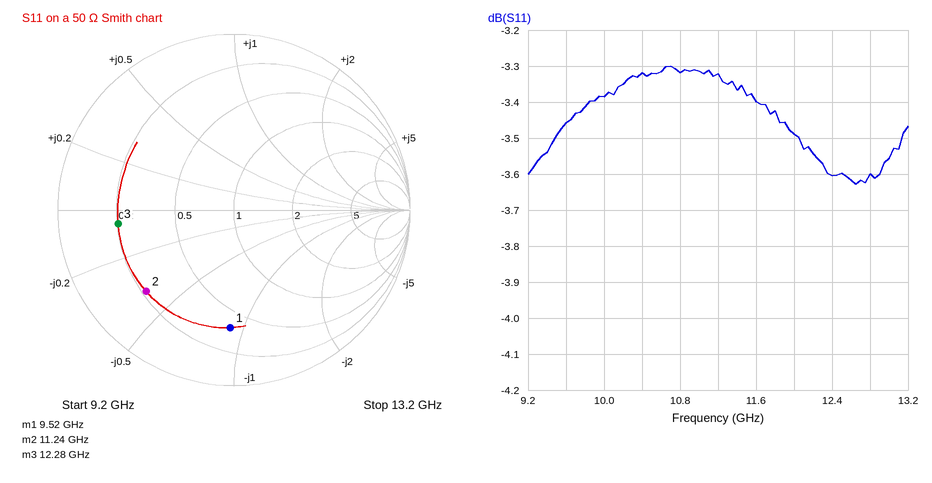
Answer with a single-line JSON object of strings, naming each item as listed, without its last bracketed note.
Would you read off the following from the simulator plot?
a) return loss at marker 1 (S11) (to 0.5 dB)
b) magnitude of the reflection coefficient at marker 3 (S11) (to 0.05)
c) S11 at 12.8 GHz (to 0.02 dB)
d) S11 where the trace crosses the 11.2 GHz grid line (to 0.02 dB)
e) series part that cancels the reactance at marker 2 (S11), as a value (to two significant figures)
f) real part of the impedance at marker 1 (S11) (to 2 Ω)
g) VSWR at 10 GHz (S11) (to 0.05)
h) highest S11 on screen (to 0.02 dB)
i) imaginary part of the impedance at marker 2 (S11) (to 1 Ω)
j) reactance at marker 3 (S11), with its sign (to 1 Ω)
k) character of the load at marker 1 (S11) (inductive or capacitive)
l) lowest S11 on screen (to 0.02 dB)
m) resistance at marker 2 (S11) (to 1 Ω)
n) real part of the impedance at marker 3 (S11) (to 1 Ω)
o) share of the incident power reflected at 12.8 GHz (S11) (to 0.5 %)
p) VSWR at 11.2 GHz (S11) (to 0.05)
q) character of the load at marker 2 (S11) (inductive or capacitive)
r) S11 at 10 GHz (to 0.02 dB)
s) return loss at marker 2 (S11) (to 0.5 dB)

{"return loss at marker 1 (S11)": "3.5 dB", "magnitude of the reflection coefficient at marker 3 (S11)": "0.65", "S11 at 12.8 GHz": "-3.60 dB", "S11 where the trace crosses the 11.2 GHz grid line": "-3.32 dB", "series part that cancels the reactance at marker 2 (S11), as a value": "270 pH", "real part of the impedance at marker 1 (S11)": "18 Ω", "VSWR at 10 GHz (S11)": "5.20", "highest S11 on screen": "-3.30 dB", "imaginary part of the impedance at marker 2 (S11)": "-19 Ω", "reactance at marker 3 (S11), with its sign": "-3 Ω", "character of the load at marker 1 (S11)": "capacitive", "lowest S11 on screen": "-3.62 dB", "resistance at marker 2 (S11)": "11 Ω", "real part of the impedance at marker 3 (S11)": "10 Ω", "share of the incident power reflected at 12.8 GHz (S11)": "43.5 %", "VSWR at 11.2 GHz (S11)": "5.30", "character of the load at marker 2 (S11)": "capacitive", "S11 at 10 GHz": "-3.38 dB", "return loss at marker 2 (S11)": "3.5 dB"}
